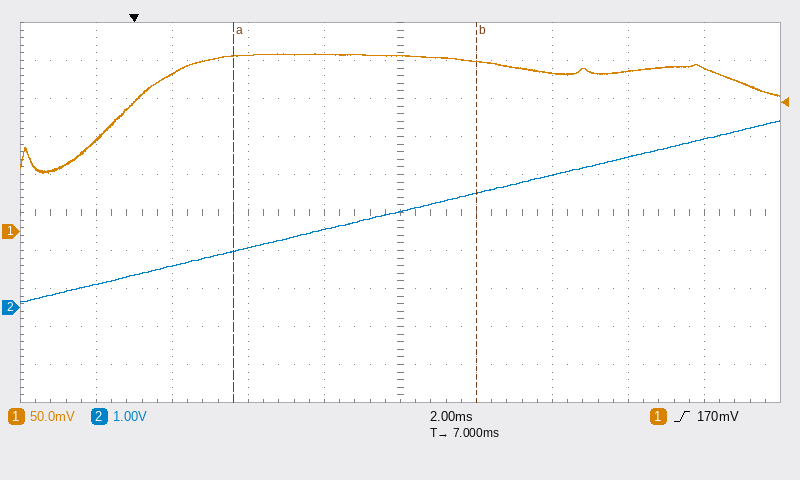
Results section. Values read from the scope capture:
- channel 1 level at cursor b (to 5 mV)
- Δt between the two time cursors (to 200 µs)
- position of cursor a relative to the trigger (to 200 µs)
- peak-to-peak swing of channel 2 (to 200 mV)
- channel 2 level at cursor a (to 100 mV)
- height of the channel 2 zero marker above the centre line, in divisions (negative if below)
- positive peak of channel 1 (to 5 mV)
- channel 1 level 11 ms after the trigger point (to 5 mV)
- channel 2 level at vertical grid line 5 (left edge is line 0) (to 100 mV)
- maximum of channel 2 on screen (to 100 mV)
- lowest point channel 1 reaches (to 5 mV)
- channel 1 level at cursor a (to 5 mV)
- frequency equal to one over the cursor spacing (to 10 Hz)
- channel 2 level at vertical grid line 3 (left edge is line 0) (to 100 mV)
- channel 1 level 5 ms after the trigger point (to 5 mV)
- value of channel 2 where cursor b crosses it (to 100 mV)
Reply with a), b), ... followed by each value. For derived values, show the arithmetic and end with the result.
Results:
a) 225 mV
b) 6.4 ms
c) +2.6 ms
d) 4.8 V
e) 1.5 V
f) -2.5 div
g) 235 mV
h) 210 mV
i) 2.5 V
j) 4.9 V
k) 75 mV
l) 230 mV
m) 1 / 6.4 ms ≈ 160 Hz
n) 1.6 V
o) 235 mV
p) 3.0 V
